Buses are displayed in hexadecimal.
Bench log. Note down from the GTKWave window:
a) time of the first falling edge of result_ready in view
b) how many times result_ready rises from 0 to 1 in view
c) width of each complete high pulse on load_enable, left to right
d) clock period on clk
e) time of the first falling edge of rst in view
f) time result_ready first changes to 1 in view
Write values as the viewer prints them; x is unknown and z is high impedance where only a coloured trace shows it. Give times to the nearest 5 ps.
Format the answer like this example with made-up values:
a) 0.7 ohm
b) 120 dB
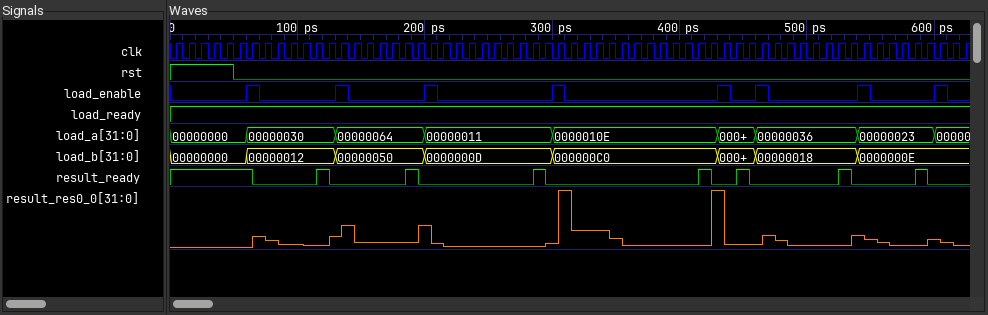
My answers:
a) 65 ps
b) 7
c) 10 ps, 10 ps, 10 ps, 10 ps, 10 ps, 10 ps, 10 ps, 10 ps
d) 10 ps
e) 50 ps
f) 115 ps
